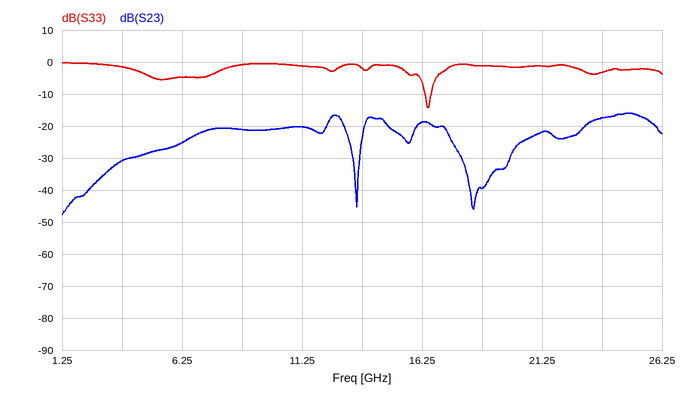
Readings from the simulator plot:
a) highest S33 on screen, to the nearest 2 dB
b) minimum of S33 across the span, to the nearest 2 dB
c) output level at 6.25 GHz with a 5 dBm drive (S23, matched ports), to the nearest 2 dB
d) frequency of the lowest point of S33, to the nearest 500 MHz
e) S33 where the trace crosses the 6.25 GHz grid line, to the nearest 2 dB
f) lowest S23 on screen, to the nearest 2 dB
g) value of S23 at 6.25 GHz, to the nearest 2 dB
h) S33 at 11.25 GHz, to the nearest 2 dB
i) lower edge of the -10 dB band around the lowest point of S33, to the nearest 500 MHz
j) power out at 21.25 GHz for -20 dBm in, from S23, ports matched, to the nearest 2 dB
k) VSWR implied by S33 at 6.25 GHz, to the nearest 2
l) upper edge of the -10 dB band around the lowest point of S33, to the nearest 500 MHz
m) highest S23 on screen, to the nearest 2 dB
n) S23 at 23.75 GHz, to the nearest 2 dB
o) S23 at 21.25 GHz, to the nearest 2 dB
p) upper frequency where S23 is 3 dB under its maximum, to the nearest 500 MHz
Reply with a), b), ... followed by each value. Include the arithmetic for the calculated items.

a) 0 dB
b) -14 dB
c) 5 dBm + (-26 dB) = -20 dBm
d) 16.5 GHz
e) -4 dB
f) -48 dB
g) -26 dB
h) -2 dB
i) 16.5 GHz
j) -20 dBm + (-22 dB) = -42 dBm
k) |Γ| = 10^(-4/20) = 0.6310; VSWR = (1 + 0.6310)/(1 − 0.6310) ≈ 4
l) 16.5 GHz
m) -16 dB
n) -18 dB
o) -22 dB
p) 26.0 GHz
